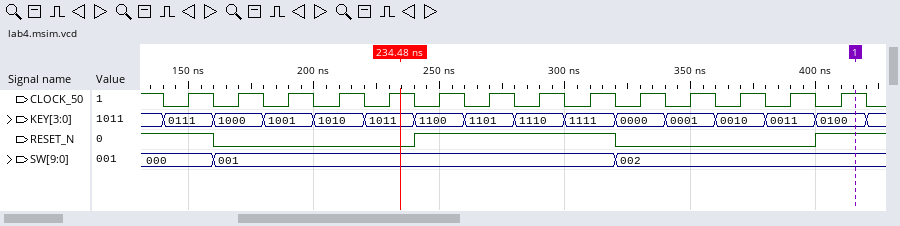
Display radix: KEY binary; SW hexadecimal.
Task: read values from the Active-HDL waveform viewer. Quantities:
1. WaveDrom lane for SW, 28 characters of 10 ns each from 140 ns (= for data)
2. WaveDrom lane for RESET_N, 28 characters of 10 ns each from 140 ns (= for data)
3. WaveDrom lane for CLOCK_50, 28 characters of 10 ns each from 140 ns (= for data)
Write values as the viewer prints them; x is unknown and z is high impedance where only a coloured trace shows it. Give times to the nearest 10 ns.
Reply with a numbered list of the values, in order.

1. {name: 'SW', wave: '=.=...............=.........', data: '000 001 002'}
2. {name: 'RESET_N', wave: '1.0.......1.......0.......1.'}
3. {name: 'CLOCK_50', wave: '0101010101010101010101010101'}
